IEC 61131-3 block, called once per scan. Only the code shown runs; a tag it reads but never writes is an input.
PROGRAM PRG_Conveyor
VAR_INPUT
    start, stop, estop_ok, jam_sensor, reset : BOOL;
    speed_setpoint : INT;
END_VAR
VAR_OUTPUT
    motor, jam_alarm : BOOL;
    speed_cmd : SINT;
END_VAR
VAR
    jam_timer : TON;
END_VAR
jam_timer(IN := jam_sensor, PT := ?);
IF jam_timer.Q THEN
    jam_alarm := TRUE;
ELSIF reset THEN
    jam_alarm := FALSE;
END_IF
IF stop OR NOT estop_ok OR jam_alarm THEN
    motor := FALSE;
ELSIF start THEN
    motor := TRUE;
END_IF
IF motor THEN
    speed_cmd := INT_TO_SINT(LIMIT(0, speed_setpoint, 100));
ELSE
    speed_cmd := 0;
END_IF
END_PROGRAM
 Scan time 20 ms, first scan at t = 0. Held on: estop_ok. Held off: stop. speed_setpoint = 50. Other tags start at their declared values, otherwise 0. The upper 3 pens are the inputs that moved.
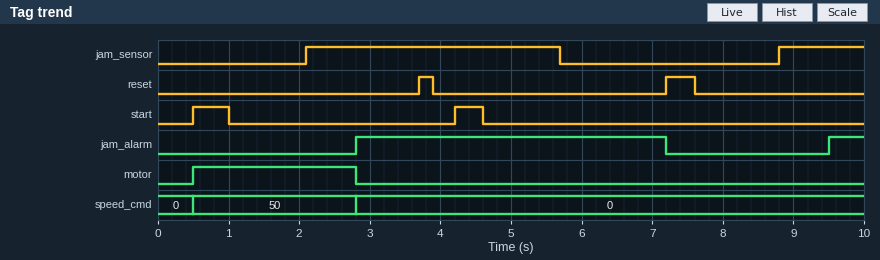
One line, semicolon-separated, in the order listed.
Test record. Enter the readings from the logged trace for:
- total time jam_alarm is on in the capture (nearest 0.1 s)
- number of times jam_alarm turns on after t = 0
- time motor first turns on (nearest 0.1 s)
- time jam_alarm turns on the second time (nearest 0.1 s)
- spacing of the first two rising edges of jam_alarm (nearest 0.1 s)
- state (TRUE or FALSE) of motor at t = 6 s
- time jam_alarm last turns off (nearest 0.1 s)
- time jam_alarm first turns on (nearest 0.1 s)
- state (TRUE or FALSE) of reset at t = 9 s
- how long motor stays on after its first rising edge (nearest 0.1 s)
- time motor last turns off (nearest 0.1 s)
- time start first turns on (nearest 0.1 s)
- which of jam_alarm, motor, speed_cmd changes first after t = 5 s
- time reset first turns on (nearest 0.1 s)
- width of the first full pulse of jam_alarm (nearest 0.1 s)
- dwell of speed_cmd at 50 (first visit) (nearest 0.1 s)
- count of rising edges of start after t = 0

4.9 s; 2; 0.5 s; 9.5 s; 6.7 s; FALSE; 7.2 s; 2.8 s; FALSE; 2.3 s; 2.8 s; 0.5 s; jam_alarm; 3.7 s; 4.4 s; 2.3 s; 2
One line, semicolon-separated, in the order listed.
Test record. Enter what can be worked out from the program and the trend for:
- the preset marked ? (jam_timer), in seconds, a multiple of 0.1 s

0.7 s
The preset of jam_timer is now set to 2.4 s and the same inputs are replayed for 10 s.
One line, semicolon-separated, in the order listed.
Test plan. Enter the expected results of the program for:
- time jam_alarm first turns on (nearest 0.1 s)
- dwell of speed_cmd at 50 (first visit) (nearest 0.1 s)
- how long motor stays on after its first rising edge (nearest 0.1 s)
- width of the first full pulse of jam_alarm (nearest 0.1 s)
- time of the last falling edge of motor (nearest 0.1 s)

4.5 s; 4.0 s; 4.0 s; 2.7 s; 4.5 s
